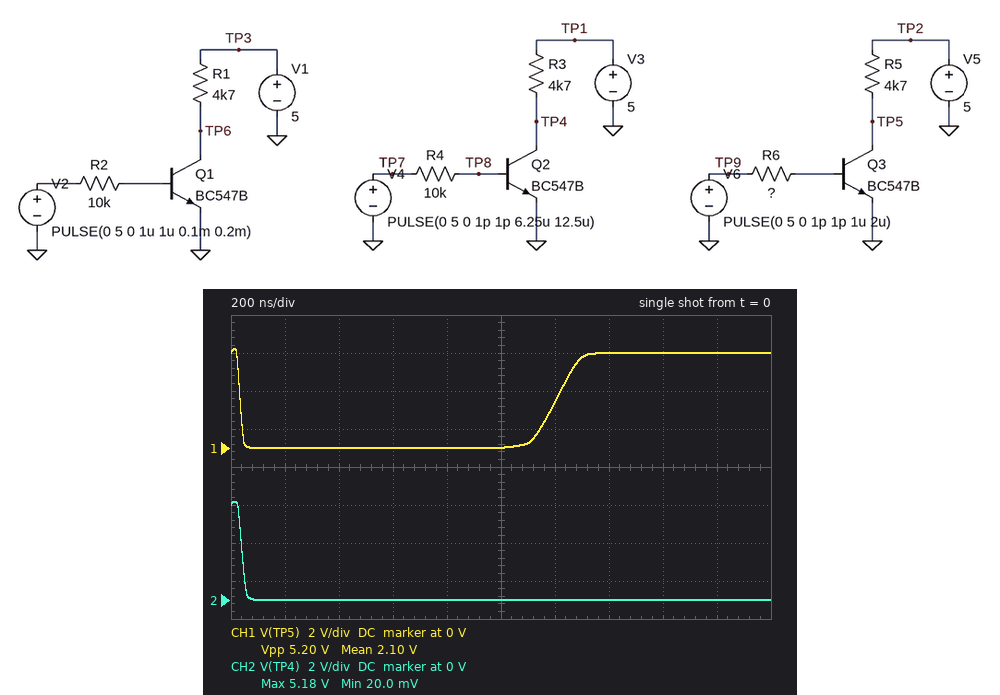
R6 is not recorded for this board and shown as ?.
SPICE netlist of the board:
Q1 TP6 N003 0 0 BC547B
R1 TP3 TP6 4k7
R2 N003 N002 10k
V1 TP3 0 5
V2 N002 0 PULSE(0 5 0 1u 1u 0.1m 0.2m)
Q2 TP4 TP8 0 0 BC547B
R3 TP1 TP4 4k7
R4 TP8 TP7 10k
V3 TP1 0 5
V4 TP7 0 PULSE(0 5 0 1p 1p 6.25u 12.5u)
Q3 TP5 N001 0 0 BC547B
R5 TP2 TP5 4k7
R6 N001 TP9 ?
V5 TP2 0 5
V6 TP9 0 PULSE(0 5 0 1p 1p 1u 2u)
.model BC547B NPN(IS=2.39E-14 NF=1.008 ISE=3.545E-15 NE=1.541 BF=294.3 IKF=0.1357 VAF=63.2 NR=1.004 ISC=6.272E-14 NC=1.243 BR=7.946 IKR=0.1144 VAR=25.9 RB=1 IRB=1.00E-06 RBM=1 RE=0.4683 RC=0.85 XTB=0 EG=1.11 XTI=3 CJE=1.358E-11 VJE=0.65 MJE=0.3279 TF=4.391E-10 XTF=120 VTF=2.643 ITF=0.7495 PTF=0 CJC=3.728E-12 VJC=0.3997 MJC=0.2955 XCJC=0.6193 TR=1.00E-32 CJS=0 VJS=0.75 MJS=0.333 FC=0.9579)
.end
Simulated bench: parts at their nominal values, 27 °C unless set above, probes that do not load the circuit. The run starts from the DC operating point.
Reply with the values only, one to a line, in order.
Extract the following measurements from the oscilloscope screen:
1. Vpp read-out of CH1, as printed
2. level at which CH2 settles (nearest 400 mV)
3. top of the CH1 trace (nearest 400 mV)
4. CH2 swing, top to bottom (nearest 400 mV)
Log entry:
5.20 V
0 V
5.2 V
5.2 V
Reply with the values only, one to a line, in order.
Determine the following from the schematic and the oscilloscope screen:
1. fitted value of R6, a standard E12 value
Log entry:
8.2 kΩ
